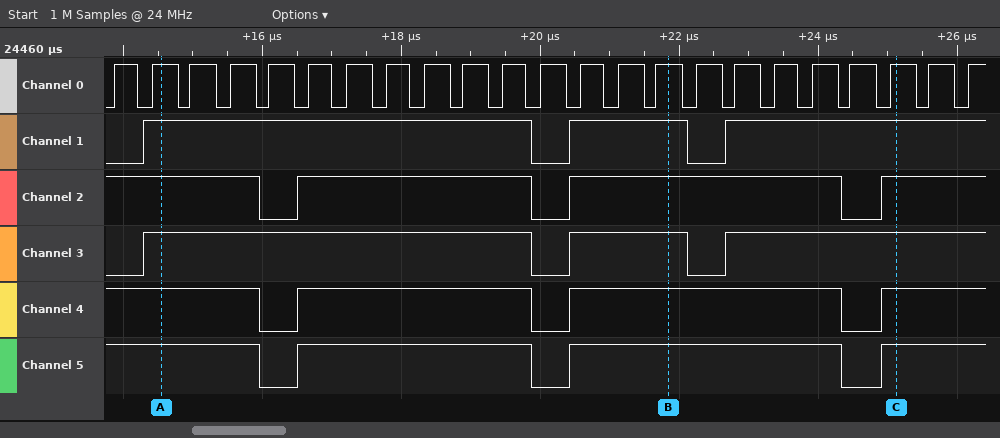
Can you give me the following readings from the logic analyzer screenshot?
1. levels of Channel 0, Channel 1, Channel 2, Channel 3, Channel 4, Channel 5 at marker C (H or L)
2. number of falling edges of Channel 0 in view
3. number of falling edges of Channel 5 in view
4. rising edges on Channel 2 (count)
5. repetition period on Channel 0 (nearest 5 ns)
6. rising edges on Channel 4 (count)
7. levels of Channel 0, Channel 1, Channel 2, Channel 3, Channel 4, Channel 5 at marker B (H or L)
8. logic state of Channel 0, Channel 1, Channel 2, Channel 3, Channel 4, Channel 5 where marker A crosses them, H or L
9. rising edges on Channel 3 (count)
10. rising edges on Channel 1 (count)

Channel 0=H, Channel 1=H, Channel 2=H, Channel 3=H, Channel 4=H, Channel 5=H
22
3
3
560 ns
3
Channel 0=H, Channel 1=H, Channel 2=H, Channel 3=H, Channel 4=H, Channel 5=H
Channel 0=H, Channel 1=H, Channel 2=H, Channel 3=H, Channel 4=H, Channel 5=H
3
3
